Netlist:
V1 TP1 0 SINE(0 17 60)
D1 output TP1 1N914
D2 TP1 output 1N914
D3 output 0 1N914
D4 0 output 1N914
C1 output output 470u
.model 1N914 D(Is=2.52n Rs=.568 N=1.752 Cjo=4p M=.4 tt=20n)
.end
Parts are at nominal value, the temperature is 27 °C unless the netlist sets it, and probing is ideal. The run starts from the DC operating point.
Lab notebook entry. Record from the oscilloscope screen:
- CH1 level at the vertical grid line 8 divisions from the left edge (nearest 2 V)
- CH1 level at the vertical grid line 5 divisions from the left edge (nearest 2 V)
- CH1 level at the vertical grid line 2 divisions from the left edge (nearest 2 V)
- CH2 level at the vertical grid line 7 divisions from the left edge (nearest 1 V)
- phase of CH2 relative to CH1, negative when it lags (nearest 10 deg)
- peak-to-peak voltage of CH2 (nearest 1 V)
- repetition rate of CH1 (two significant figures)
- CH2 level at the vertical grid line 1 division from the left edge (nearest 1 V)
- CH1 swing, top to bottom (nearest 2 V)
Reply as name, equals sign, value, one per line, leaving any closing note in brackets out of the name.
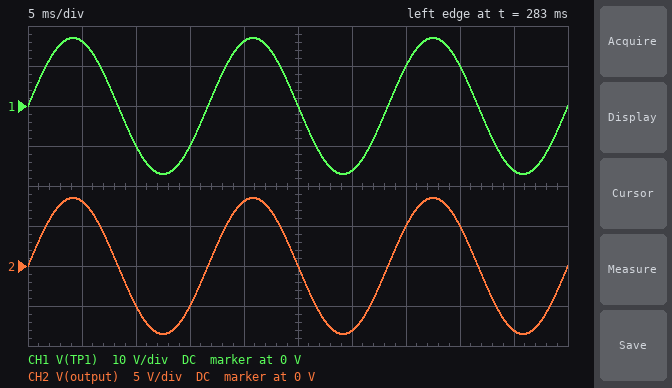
CH1 level at the vertical grid line 8 divisions from the left edge = 10 V
CH1 level at the vertical grid line 5 divisions from the left edge = 0 V
CH1 level at the vertical grid line 2 divisions from the left edge = -10 V
CH2 level at the vertical grid line 7 divisions from the left edge = 5 V
phase of CH2 relative to CH1, negative when it lags = 0 deg
peak-to-peak voltage of CH2 = 17 V
repetition rate of CH1 = 60 Hz
CH2 level at the vertical grid line 1 division from the left edge = 8 V
CH1 swing, top to bottom = 34 V
